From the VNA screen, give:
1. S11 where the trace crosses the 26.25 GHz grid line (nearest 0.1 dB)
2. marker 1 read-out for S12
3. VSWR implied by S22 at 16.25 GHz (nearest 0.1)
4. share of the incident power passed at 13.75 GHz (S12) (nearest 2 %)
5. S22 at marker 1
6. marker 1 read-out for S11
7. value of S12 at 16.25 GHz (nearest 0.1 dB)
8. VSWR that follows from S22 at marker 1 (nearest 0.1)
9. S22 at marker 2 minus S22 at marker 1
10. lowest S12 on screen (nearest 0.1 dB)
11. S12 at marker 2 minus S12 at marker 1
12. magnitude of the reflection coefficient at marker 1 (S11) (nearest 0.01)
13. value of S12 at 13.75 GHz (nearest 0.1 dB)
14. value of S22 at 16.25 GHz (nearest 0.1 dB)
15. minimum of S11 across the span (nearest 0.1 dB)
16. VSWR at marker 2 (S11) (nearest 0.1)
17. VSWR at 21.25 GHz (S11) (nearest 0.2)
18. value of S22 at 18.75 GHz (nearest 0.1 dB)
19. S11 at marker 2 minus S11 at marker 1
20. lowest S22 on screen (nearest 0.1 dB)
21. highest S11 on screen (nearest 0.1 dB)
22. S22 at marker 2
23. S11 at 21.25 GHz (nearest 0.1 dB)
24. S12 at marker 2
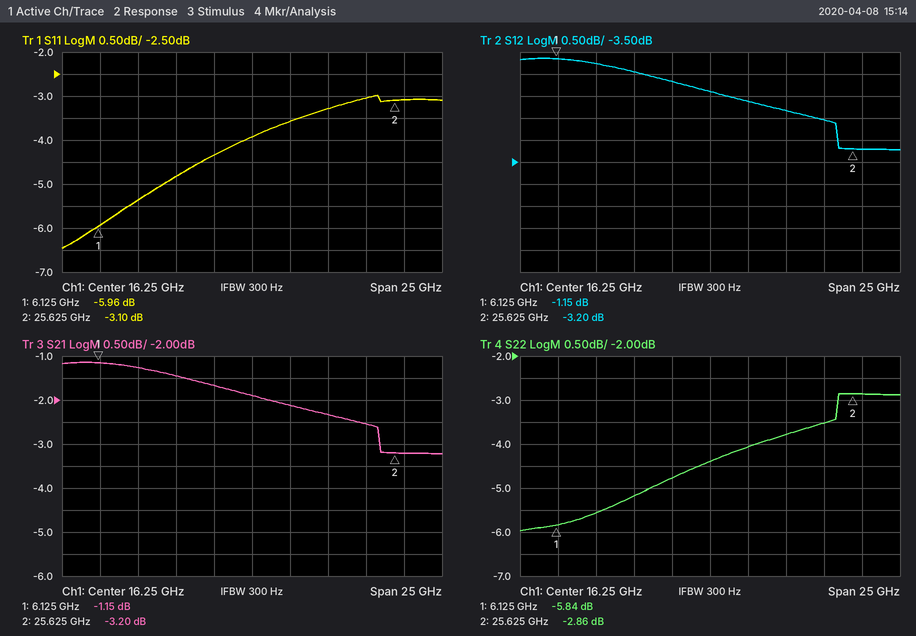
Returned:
-3.1 dB
-1.15 dB
4.0
68 %
-5.84 dB
-5.96 dB
-1.9 dB
3.1
2.98 dB
-3.2 dB
-2.05 dB
0.50
-1.7 dB
-4.4 dB
-6.5 dB
5.7
5.4
-4.1 dB
2.86 dB
-6.0 dB
-3.0 dB
-2.86 dB
-3.3 dB
-3.20 dB
